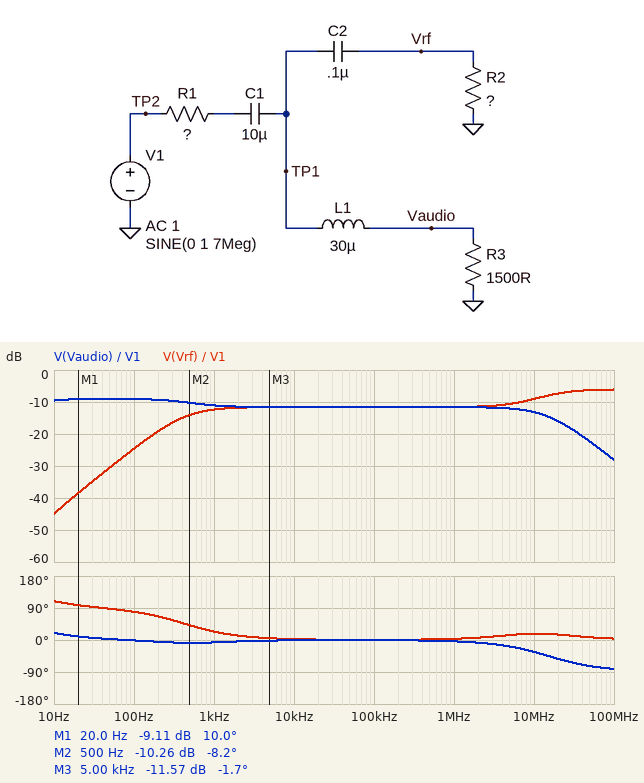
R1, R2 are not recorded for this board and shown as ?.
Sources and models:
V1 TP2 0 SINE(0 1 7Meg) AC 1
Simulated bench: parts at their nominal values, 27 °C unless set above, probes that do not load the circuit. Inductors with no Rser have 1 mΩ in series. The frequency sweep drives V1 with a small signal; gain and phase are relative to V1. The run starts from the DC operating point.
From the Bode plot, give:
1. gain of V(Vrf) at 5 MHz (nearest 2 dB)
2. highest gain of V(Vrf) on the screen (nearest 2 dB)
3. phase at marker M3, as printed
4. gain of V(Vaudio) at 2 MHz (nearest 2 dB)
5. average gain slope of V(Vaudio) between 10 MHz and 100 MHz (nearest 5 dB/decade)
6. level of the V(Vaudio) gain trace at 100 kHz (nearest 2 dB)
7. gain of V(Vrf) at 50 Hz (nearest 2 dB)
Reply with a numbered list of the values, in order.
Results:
1. -10 dB
2. -6 dB
3. -1.7 deg
4. -12 dB
5. -15 dB/decade
6. -12 dB
7. -30 dB
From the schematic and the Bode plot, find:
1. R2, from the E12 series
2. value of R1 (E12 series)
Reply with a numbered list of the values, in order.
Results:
1. 2.7 kΩ
2. 2.7 kΩ
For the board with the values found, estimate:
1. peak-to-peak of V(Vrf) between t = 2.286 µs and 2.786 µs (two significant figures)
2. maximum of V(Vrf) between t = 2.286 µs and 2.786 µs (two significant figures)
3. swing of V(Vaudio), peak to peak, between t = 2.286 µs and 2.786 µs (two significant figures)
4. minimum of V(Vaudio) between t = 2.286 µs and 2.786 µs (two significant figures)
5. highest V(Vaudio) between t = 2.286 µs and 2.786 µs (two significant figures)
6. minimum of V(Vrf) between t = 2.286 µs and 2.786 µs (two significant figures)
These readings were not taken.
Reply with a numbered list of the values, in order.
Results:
1. 640 mV
2. 320 mV
3. 480 mV
4. -240 mV
5. 240 mV
6. -320 mV
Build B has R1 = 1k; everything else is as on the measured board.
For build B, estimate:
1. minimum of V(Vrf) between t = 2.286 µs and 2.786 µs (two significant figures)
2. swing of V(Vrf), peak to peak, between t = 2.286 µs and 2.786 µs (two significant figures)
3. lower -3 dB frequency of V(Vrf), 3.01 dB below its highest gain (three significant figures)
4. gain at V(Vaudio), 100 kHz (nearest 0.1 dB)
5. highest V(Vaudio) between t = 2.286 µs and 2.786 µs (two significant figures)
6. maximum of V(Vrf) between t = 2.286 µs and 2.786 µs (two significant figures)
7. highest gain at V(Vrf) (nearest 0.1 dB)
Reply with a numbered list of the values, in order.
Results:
1. -560 mV
2. 1.1 V
3. 3.64 MHz
4. -6.2 dB
5. 420 mV
6. 560 mV
7. -2.7 dB
